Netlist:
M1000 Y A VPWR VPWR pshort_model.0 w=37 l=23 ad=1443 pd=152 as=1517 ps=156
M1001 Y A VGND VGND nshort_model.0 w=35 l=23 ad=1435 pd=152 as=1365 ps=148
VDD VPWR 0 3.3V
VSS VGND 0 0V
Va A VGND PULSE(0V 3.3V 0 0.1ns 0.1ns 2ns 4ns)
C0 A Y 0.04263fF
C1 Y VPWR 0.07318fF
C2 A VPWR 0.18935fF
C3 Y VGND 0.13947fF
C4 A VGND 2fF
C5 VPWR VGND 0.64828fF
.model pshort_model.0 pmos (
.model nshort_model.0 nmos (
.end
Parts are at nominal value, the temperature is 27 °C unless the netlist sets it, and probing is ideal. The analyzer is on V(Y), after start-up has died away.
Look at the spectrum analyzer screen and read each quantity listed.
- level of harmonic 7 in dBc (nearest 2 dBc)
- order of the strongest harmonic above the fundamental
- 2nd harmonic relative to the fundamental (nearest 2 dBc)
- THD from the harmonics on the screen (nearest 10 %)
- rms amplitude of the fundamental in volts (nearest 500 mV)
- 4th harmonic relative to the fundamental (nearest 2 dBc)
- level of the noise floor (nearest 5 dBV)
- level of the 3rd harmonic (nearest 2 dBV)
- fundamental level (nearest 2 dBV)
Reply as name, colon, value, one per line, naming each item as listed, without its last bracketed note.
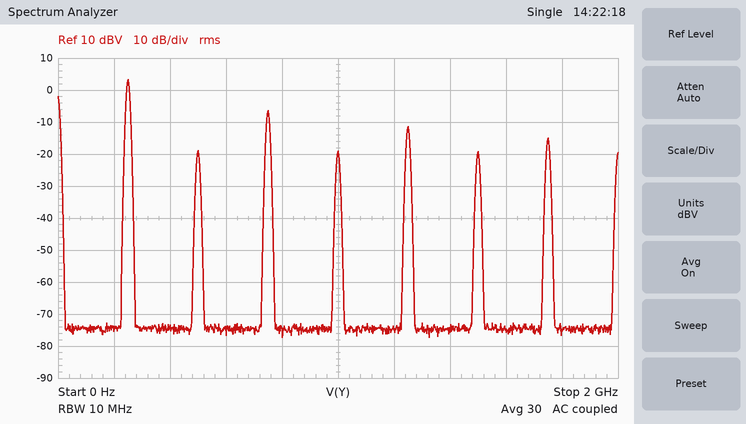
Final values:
level of harmonic 7 in dBc: -18 dBc
order of the strongest harmonic above the fundamental: 3
2nd harmonic relative to the fundamental: -22 dBc
THD from the harmonics on the screen: 40 %
rms amplitude of the fundamental in volts: 1.5 V
4th harmonic relative to the fundamental: -22 dBc
level of the noise floor: -75 dBV
level of the 3rd harmonic: -6 dBV
fundamental level: 4 dBV
